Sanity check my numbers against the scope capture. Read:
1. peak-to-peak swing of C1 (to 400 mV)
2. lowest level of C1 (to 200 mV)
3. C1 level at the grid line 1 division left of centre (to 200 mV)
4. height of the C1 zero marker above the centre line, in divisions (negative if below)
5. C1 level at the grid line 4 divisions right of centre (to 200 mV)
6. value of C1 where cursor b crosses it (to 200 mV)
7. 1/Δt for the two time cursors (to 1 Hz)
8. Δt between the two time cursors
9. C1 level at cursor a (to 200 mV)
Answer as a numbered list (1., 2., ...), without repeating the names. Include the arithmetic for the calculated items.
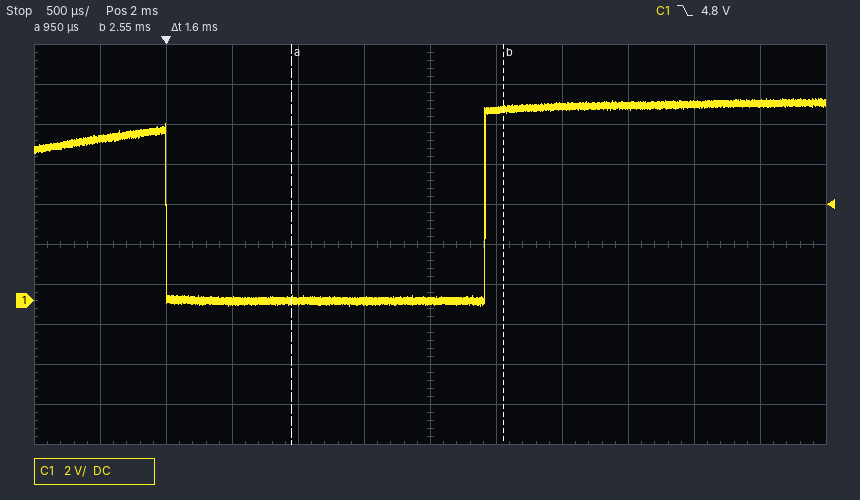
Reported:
1. 10.4 V
2. -200 mV
3. 0.0 V
4. -1.4 div
5. 9.8 V
6. 9.6 V
7. 1 / 1.6 ms ≈ 625 Hz
8. 1.6 ms
9. 0.0 V
